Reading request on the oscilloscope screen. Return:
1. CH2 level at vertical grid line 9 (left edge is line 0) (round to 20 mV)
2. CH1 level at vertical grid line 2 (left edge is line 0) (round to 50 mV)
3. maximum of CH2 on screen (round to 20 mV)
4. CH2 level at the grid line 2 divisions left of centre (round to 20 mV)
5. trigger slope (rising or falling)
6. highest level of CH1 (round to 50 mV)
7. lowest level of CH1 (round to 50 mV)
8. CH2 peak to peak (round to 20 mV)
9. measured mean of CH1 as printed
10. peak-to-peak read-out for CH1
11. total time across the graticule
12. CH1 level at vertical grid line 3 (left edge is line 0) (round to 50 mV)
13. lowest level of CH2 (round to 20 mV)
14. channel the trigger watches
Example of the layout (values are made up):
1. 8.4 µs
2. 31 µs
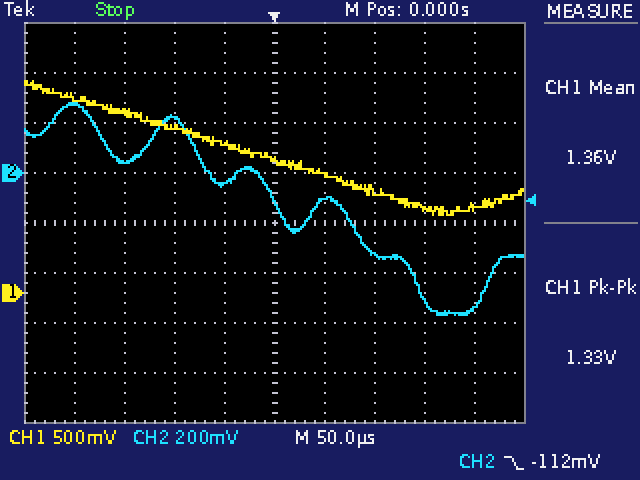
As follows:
1. -540 mV
2. 1.80 V
3. 280 mV
4. 220 mV
5. falling
6. 2.10 V
7. 800 mV
8. 840 mV
9. 1.36 V
10. 1.33 V
11. 500 µs
12. 1.65 V
13. -560 mV
14. CH2
